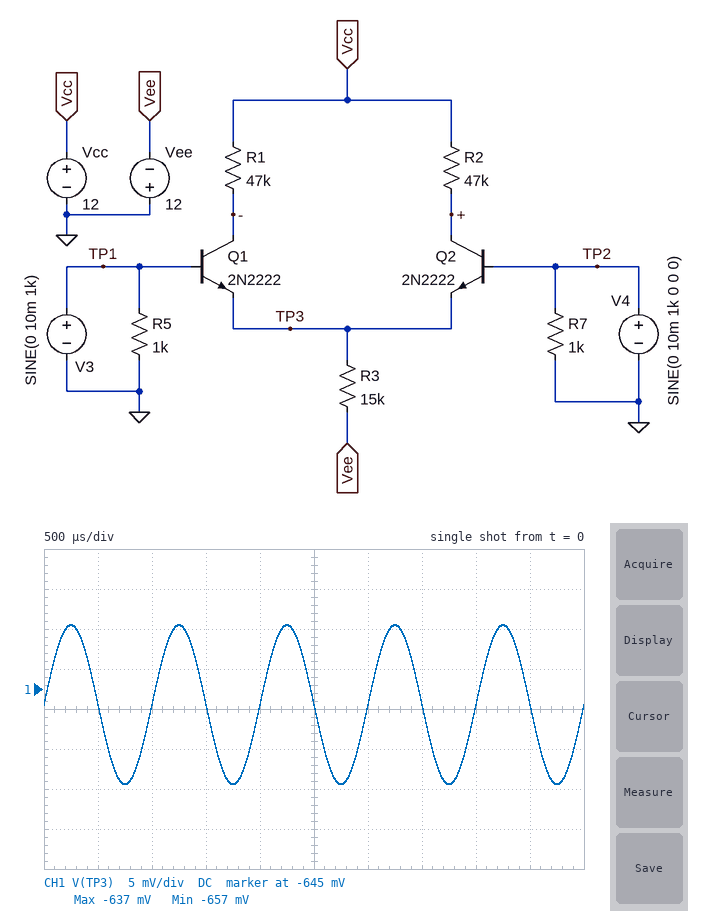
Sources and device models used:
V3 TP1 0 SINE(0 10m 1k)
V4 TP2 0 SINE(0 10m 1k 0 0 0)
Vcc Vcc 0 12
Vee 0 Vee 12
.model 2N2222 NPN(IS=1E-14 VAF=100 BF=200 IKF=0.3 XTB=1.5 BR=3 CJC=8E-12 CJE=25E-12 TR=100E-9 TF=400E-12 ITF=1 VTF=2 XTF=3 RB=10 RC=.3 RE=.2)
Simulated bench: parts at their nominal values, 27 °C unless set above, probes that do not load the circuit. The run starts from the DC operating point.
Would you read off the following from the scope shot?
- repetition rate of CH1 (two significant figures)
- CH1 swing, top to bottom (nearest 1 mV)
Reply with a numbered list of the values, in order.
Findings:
1. 1.0 kHz
2. 20 mV
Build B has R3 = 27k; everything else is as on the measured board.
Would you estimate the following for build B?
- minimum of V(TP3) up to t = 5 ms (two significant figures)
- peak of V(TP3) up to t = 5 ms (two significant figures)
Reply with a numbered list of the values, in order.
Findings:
1. -620 mV
2. -600 mV
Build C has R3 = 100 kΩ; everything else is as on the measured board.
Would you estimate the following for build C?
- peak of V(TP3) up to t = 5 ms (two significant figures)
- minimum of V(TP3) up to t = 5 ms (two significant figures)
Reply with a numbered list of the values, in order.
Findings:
1. -570 mV
2. -590 mV
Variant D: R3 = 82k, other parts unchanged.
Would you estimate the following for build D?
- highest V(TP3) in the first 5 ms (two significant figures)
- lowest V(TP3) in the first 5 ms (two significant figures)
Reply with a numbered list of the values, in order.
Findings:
1. -570 mV
2. -590 mV
